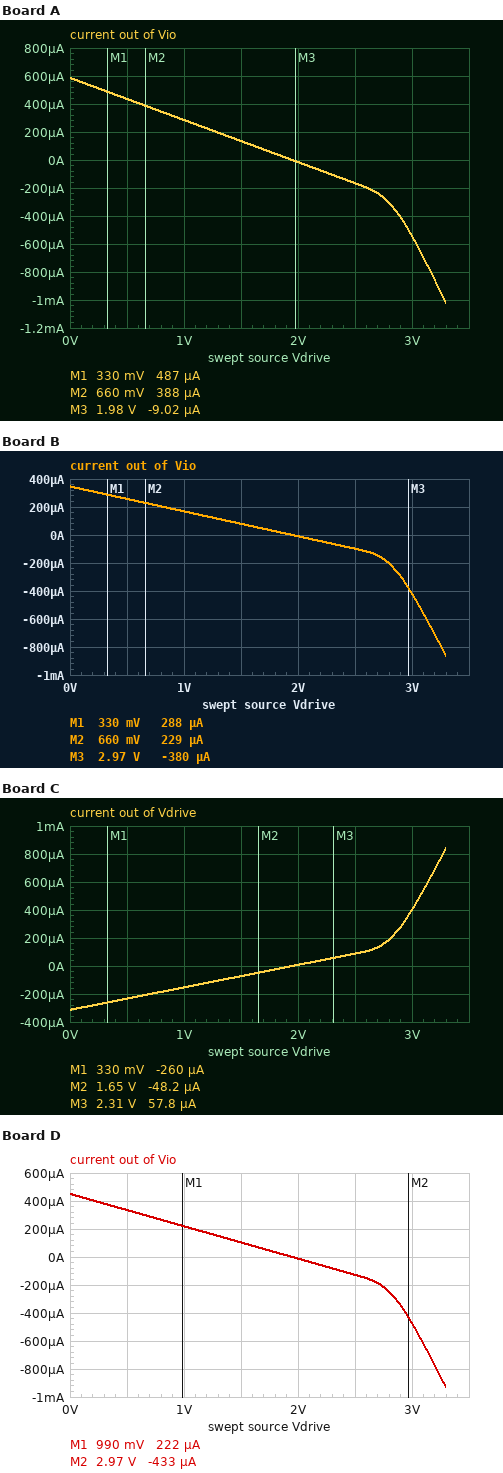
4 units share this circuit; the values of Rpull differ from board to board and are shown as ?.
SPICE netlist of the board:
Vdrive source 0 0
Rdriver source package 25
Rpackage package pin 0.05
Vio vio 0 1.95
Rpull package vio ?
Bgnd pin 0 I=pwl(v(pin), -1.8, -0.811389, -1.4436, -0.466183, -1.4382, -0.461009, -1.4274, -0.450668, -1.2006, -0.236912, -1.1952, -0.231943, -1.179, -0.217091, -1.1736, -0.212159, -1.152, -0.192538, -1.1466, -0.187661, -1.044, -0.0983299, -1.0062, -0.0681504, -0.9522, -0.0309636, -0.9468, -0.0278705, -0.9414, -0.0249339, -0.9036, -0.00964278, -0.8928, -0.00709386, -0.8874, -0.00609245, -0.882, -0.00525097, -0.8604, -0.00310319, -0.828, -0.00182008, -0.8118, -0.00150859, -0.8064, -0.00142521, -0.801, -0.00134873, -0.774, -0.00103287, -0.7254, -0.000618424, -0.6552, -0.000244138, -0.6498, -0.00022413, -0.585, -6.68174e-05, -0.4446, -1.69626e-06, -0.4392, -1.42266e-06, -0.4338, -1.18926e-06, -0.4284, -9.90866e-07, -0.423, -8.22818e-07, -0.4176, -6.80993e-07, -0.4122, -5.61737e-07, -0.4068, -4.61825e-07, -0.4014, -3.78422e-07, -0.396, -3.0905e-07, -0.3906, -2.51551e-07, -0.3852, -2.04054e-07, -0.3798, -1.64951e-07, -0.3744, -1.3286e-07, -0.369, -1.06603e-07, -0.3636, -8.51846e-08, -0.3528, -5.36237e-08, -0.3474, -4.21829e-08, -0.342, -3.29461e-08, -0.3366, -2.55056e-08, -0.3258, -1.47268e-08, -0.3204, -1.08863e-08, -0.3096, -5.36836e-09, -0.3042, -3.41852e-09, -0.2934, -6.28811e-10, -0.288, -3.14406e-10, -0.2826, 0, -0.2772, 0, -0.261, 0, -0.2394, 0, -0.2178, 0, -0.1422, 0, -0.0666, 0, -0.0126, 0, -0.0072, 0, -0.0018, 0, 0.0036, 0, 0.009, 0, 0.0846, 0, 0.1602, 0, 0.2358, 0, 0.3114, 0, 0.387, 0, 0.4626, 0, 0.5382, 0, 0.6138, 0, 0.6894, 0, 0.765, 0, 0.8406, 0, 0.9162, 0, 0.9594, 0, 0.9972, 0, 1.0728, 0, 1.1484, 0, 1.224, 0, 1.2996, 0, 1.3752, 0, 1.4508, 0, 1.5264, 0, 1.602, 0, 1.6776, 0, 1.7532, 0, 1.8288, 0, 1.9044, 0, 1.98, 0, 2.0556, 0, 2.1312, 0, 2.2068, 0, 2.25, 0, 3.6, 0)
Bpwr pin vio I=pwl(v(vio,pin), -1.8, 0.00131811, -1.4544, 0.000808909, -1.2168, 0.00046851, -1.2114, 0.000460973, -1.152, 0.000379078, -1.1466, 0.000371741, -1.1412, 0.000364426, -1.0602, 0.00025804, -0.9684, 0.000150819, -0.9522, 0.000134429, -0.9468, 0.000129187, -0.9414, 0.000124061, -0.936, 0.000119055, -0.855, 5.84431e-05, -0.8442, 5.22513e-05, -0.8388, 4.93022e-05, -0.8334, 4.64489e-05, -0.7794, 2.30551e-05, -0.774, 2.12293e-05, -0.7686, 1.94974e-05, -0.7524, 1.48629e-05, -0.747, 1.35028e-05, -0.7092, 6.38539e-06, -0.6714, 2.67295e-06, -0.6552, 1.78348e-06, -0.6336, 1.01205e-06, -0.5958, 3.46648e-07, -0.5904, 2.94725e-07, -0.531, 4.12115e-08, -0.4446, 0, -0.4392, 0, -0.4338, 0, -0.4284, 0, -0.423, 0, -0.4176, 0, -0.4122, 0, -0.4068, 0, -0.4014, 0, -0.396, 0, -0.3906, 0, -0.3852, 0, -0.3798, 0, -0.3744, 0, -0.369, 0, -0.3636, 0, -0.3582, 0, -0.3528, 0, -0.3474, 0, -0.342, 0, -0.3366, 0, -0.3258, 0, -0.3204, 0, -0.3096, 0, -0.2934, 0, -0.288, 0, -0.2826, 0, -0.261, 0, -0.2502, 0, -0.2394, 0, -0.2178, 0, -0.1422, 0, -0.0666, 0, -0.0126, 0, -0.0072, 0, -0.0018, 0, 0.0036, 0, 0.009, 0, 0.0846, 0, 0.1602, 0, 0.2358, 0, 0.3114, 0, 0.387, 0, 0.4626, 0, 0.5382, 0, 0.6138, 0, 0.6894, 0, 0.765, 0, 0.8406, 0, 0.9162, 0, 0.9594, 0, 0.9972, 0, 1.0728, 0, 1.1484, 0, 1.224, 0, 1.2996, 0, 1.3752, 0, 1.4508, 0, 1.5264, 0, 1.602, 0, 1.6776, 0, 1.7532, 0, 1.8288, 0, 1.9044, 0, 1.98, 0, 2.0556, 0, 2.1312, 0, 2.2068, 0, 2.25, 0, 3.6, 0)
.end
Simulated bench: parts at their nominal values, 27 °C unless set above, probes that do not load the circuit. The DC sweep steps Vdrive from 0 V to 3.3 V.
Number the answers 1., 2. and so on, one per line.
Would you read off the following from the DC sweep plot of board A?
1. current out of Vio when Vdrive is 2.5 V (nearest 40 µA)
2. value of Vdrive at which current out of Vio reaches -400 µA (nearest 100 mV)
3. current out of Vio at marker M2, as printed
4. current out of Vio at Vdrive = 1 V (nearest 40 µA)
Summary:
1. -160 µA
2. 2.9 V
3. 388 µA
4. 280 µA
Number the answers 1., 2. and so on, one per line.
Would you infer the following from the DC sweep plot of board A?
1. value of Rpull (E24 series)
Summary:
1. 3.3 kΩ
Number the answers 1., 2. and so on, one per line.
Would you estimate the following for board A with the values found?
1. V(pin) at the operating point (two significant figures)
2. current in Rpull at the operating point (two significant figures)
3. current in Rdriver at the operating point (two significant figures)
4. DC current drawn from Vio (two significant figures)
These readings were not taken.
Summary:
1. 15 mV
2. 590 µA
3. 590 µA
4. 590 µA
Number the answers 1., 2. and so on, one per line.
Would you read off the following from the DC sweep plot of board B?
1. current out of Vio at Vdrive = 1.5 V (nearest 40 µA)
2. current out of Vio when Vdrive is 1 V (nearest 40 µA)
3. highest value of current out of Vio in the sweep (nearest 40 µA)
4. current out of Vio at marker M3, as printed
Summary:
1. 80 µA
2. 160 µA
3. 360 µA
4. -380 µA
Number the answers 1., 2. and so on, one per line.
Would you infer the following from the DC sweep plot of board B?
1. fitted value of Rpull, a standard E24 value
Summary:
1. 5.6 kΩ
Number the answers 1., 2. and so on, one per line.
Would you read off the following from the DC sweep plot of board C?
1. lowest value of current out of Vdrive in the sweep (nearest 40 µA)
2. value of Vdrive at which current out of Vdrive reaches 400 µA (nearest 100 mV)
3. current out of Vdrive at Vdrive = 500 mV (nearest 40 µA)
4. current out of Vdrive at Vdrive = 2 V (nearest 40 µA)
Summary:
1. -320 µA
2. 3.0 V
3. -240 µA
4. 0 A
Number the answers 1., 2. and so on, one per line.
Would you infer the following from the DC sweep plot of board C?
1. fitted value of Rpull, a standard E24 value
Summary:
1. 6.2 kΩ
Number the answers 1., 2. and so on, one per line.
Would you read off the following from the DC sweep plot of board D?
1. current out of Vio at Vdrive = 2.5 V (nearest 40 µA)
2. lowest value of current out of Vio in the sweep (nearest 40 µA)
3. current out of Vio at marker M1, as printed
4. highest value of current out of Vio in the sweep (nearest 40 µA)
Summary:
1. -120 µA
2. -920 µA
3. 222 µA
4. 440 µA
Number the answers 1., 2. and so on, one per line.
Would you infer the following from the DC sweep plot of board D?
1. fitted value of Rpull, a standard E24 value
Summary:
1. 4.3 kΩ
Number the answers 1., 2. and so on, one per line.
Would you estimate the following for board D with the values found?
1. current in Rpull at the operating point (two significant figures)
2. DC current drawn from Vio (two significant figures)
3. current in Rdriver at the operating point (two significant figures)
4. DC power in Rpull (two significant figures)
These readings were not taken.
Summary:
1. 450 µA
2. 450 µA
3. 450 µA
4. 870 µW
